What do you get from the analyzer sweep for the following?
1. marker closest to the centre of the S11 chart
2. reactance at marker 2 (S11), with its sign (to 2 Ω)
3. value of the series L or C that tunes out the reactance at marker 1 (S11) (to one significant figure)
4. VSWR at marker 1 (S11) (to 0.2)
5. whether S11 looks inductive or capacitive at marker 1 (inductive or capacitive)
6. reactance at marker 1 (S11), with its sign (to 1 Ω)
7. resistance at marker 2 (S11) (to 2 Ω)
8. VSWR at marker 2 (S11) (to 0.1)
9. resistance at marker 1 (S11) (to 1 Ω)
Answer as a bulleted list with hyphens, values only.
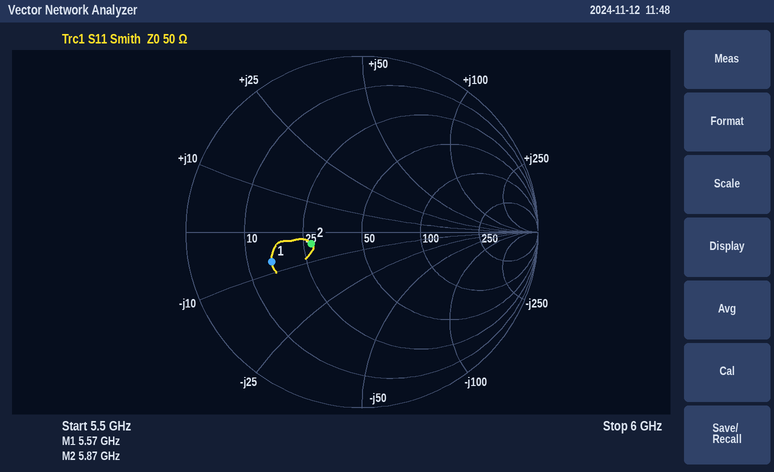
- marker 2
- -4 Ω
- 200 pH
- 3.4
- capacitive
- -7 Ω
- 28 Ω
- 1.8
- 15 Ω
